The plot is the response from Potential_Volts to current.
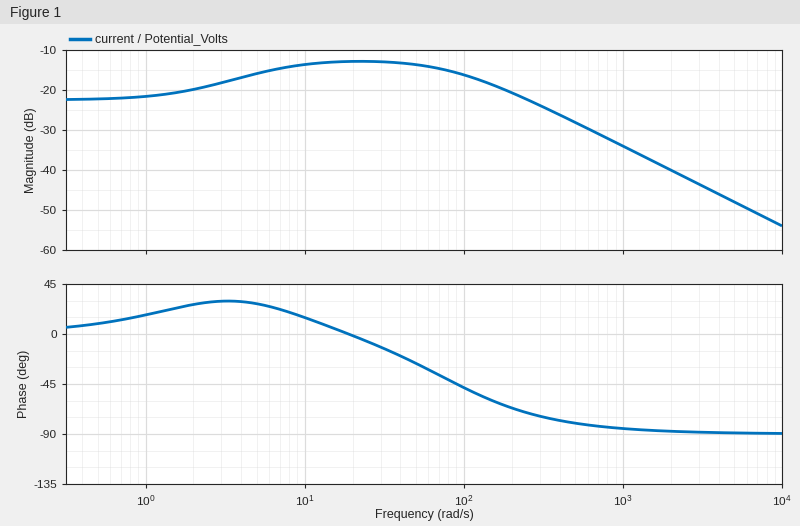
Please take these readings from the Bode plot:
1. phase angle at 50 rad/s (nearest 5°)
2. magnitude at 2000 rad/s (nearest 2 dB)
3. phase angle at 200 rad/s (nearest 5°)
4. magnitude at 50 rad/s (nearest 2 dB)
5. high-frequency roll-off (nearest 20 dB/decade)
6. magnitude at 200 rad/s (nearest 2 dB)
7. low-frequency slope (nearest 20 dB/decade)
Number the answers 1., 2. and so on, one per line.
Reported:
1. -25°
2. -40 dB
3. -65°
4. -14 dB
5. -20 dB/decade
6. -20 dB
7. 0 dB/decade
